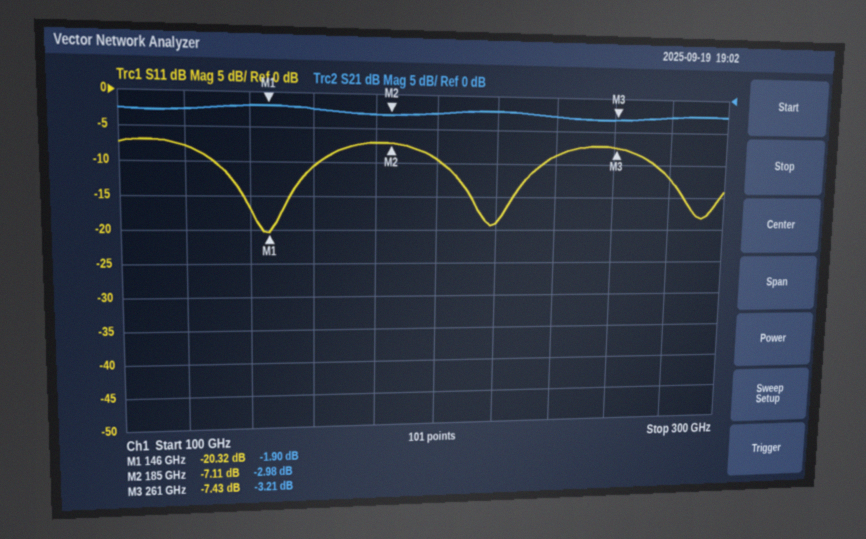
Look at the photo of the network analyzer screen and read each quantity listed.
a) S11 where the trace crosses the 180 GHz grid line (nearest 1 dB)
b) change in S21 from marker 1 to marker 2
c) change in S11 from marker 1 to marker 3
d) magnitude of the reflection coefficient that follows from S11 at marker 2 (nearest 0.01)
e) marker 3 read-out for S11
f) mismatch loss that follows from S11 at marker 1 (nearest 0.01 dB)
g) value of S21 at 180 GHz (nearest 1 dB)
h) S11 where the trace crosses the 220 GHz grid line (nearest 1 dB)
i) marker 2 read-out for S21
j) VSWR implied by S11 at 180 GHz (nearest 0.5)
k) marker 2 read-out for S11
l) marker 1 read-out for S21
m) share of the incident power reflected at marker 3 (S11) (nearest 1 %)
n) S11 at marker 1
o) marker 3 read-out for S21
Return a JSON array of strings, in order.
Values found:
["-7 dB", "-1.08 dB", "12.89 dB", "0.44", "-7.43 dB", "0.04 dB", "-3 dB", "-19 dB", "-2.98 dB", "2.5", "-7.11 dB", "-1.90 dB", "18 %", "-20.32 dB", "-3.21 dB"]
